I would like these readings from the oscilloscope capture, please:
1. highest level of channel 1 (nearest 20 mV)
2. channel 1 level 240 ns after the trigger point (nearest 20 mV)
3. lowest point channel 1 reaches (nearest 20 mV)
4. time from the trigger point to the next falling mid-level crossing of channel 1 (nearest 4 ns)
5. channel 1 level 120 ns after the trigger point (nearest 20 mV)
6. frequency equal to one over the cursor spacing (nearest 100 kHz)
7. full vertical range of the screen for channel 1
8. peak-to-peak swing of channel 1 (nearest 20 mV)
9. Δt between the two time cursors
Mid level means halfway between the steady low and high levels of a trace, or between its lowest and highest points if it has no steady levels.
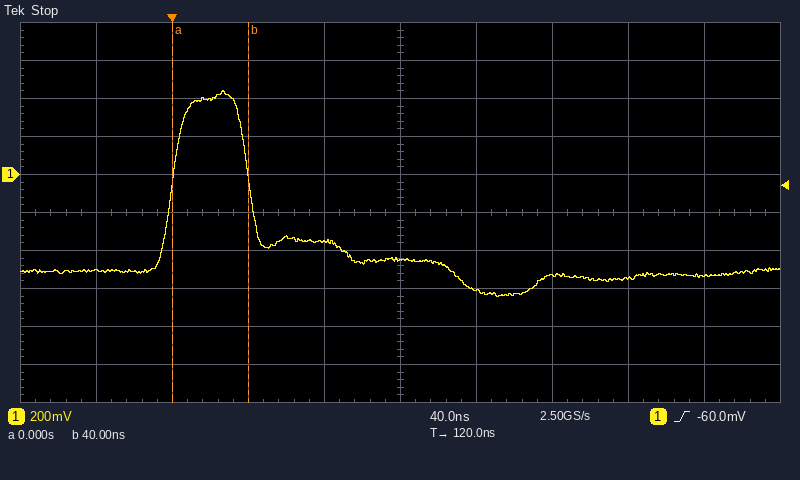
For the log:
440 mV
-540 mV
-640 mV
40 ns
-440 mV
25.0 MHz
2 V
1.08 V
40 ns
